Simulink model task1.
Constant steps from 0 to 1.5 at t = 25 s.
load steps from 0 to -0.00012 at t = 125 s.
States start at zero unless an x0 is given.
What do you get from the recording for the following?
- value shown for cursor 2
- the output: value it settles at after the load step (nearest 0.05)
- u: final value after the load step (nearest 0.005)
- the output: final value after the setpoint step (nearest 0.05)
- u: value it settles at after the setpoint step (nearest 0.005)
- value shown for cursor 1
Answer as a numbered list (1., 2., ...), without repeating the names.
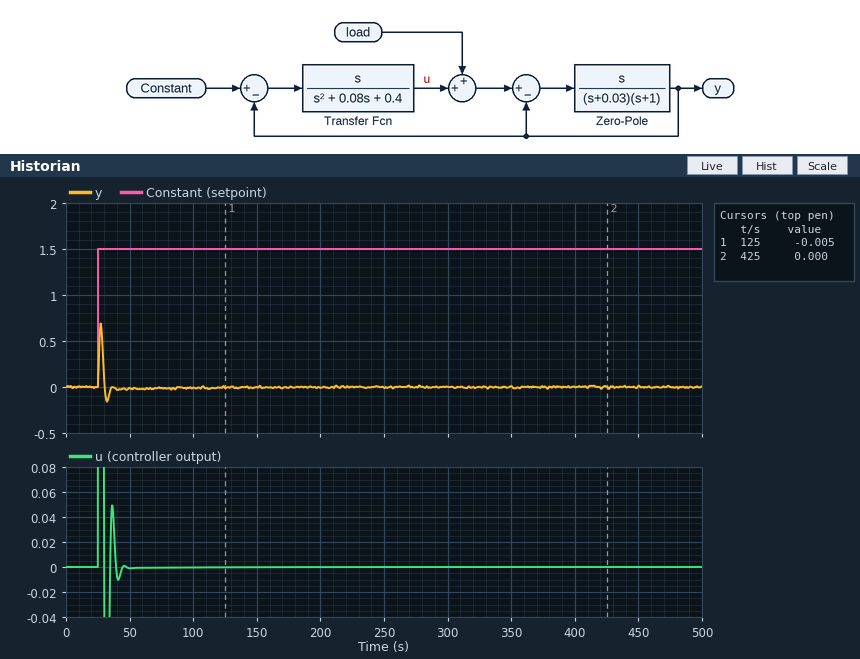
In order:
1. 0.000
2. 0.00
3. 0.000
4. 0.00
5. 0.000
6. -0.005
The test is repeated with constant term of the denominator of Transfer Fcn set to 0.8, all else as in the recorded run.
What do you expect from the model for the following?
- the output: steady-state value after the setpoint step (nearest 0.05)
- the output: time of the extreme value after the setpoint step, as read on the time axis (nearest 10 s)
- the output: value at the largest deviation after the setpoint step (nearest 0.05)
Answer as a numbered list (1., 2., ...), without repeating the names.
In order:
1. 0.00
2. 30 s
3. 0.55
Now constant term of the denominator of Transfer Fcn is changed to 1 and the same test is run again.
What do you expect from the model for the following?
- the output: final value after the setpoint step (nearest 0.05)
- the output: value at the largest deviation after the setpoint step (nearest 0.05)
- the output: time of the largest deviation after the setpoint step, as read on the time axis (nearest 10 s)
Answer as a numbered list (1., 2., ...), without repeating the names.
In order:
1. 0.00
2. 0.50
3. 30 s
